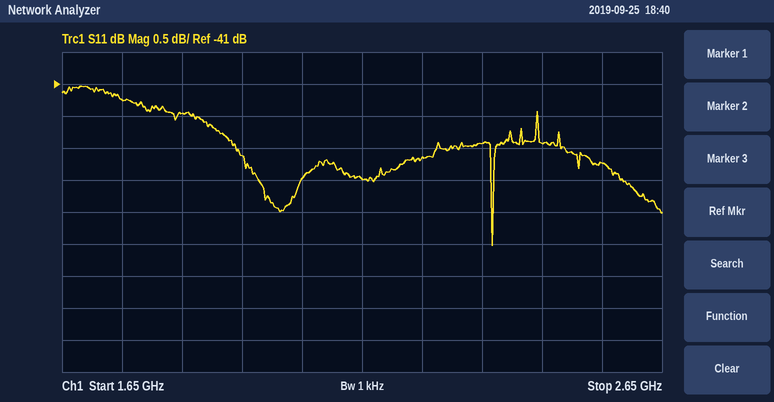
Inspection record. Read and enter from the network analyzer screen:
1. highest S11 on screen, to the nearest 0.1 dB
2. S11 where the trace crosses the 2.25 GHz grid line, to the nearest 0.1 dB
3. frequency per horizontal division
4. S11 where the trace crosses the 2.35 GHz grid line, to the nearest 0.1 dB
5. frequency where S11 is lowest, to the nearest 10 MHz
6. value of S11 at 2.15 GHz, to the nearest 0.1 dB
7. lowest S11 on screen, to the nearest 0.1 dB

-41.0 dB
-42.1 dB
100 MHz
-41.9 dB
2.37 GHz
-42.5 dB
-43.5 dB
